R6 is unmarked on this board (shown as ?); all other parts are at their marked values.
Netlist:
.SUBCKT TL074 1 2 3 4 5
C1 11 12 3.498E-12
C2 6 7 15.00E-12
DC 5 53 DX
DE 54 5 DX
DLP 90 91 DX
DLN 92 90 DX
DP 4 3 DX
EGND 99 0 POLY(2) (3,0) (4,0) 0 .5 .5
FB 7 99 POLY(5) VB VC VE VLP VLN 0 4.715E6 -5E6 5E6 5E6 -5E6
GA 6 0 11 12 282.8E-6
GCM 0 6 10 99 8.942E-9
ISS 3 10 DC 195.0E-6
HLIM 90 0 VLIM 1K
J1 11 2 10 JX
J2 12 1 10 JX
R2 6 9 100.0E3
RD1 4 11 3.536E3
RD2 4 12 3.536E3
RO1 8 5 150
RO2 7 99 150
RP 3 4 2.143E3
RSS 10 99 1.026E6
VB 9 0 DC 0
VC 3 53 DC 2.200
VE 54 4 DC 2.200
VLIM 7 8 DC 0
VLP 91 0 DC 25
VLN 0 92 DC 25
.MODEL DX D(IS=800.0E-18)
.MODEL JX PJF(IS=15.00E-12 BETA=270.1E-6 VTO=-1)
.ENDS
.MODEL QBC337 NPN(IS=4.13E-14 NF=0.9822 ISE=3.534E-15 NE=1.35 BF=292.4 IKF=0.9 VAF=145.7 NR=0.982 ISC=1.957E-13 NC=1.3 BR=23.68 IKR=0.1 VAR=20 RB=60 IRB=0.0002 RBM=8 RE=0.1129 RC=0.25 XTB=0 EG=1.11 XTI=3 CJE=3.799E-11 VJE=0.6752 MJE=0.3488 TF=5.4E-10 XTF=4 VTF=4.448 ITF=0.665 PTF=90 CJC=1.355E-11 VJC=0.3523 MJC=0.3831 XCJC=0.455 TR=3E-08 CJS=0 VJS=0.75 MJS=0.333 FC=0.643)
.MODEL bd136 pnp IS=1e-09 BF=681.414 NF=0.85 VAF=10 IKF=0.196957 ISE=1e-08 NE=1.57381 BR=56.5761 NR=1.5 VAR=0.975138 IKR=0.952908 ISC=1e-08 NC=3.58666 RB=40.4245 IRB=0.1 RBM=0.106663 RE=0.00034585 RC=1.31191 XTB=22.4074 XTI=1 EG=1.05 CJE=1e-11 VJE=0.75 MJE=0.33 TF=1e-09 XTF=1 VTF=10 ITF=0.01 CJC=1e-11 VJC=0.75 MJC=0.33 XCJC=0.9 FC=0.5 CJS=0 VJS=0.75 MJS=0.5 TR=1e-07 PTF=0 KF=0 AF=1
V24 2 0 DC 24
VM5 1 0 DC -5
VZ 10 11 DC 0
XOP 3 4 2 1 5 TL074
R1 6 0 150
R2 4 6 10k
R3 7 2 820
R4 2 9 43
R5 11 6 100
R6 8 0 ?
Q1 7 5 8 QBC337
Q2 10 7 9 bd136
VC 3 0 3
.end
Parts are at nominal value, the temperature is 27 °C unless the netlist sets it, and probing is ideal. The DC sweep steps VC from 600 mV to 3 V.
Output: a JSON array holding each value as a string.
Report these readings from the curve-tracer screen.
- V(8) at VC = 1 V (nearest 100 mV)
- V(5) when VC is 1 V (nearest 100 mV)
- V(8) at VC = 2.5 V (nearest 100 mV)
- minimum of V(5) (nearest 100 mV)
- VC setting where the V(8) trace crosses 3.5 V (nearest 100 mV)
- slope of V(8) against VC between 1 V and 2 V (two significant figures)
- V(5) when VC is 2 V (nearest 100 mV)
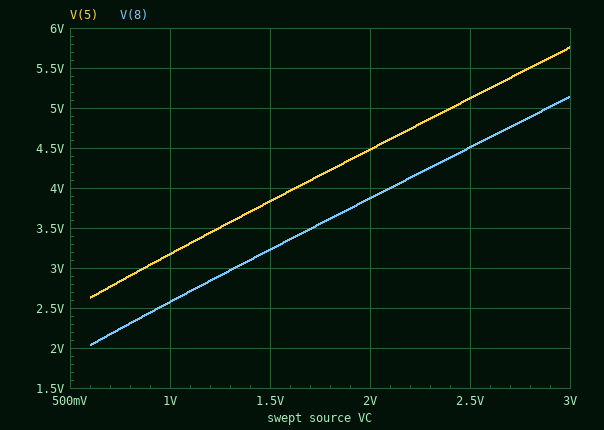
["2.6 V", "3.2 V", "4.5 V", "2.6 V", "1.7 V", "1.3 V/V", "4.5 V"]
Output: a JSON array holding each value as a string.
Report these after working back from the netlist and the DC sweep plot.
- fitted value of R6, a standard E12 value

["3.3 kΩ"]
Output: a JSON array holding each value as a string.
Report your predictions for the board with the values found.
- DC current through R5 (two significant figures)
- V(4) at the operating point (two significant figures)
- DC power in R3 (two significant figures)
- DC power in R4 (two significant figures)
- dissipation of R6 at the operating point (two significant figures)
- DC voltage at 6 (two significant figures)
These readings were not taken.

["20 mA", "3.0 V", "1.8 mW", "17 mW", "8.0 mW", "3.0 V"]
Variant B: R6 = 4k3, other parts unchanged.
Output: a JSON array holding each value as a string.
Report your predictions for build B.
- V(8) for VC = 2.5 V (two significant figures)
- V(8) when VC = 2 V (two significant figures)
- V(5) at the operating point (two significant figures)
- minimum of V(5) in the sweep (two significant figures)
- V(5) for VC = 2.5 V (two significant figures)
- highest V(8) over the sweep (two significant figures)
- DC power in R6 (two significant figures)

["5.9 V", "5.0 V", "7.3 V", "3.2 V", "6.5 V", "6.7 V", "10 mW"]
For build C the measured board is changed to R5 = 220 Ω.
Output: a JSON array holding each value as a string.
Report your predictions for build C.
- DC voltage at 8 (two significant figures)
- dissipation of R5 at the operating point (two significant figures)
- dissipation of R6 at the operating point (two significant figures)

["5.2 V", "88 mW", "8.1 mW"]
